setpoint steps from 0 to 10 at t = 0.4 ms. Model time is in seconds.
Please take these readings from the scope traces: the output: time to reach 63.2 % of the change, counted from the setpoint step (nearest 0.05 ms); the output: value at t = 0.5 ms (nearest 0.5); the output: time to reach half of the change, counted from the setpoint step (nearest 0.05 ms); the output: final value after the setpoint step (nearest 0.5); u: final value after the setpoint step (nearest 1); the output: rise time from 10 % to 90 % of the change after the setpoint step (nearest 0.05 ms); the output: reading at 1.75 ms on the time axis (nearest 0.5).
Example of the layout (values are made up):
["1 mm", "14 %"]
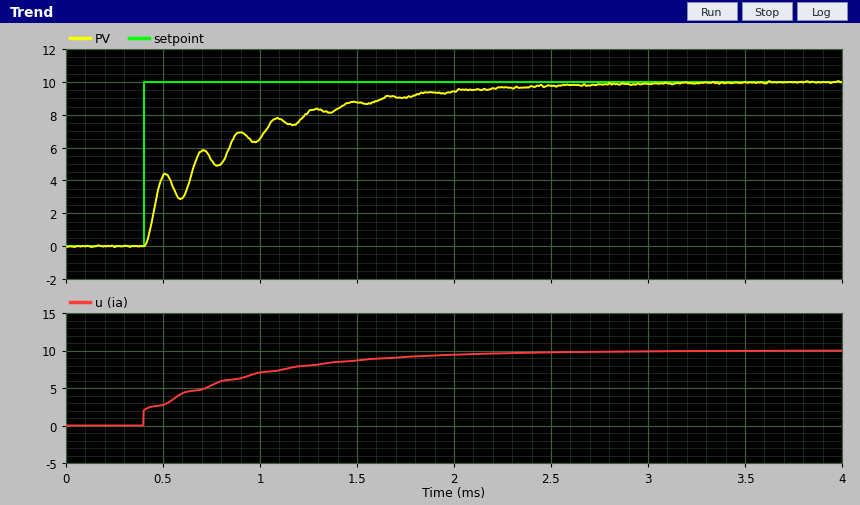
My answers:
["0.45 ms", "4.5", "0.25 ms", "10.0", "10", "1.20 ms", "9.0"]
